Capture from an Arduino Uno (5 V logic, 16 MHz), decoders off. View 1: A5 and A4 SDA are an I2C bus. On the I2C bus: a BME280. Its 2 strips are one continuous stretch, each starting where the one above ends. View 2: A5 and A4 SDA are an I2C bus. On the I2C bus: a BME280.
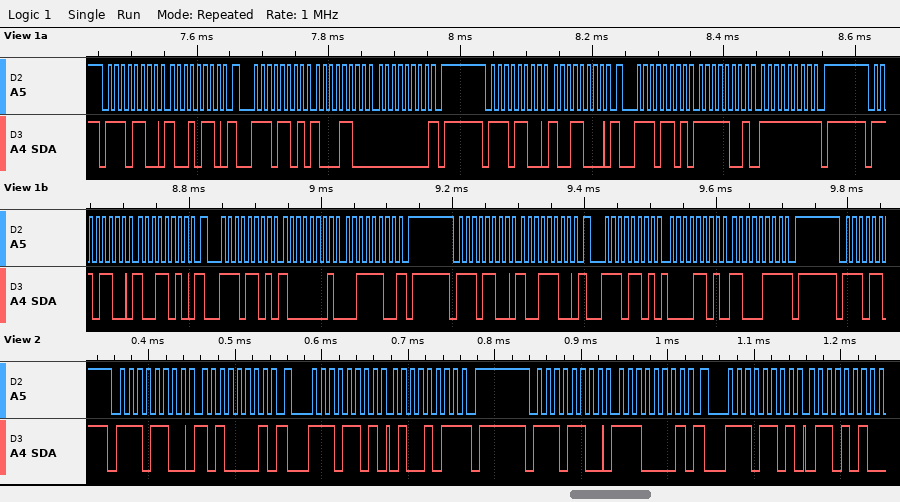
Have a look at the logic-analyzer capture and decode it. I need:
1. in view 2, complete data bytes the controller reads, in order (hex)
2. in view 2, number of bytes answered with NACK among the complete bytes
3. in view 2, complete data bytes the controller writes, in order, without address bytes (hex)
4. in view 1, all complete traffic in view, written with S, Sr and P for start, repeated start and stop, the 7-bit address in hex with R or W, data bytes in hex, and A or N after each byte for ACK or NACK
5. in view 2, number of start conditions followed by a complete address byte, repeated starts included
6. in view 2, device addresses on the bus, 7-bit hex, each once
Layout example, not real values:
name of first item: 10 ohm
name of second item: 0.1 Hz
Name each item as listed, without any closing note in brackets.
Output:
in view 2, complete data bytes the controller reads, in order: 4B 6A
in view 2, number of bytes answered with NACK among the complete bytes: 1
in view 2, complete data bytes the controller writes, in order, without address bytes: A1 E1
in view 1, all complete traffic in view, written with S, Sr and P for start, repeated start and stop, the 7-bit address in hex with R or W, data bytes in hex, and A or N after each byte for ACK or NACK: S 76W A 96 A Sr 76R A 8C A 00 N P S 76W A 98 A Sr 76R A F9 A FF N P S 76W A 9A A Sr 76R A 81 A 3C N P S 76W A 9C A Sr 76R A 0D A C7 N P
in view 2, number of start conditions followed by a complete address byte, repeated starts included: 4
in view 2, device addresses on the bus, 7-bit hex, each once: 0x76
